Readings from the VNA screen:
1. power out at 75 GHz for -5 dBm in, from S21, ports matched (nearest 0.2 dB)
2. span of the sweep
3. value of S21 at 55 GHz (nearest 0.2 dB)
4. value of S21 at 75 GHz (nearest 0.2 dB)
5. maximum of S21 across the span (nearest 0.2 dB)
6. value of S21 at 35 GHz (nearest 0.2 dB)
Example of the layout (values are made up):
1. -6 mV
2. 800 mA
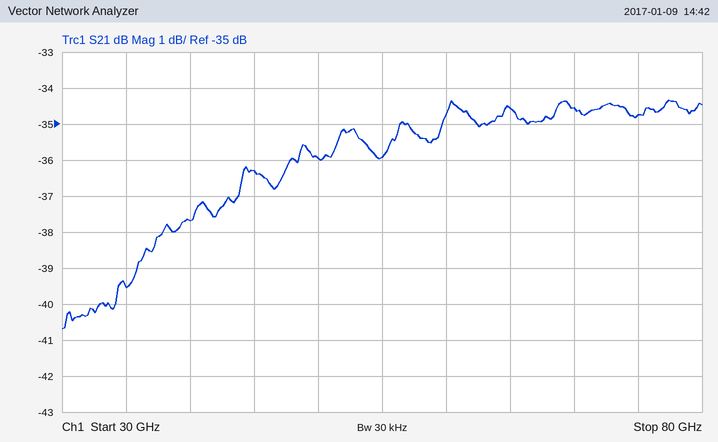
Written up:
1. -39.8 dBm
2. 50 GHz
3. -36.0 dB
4. -34.8 dB
5. -34.4 dB
6. -39.6 dB
